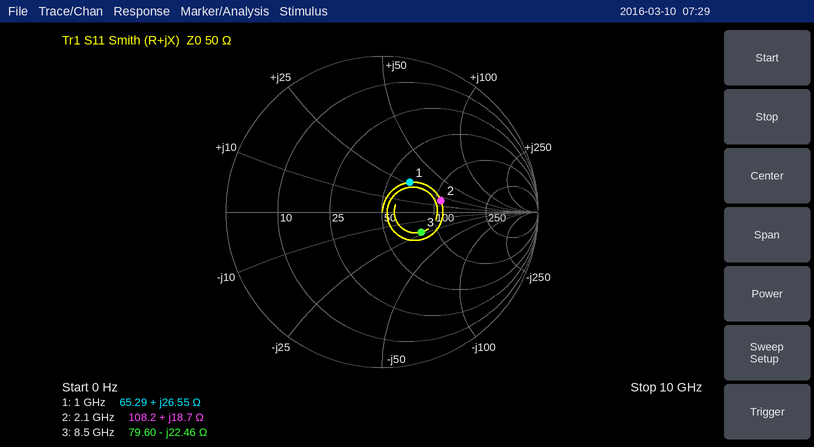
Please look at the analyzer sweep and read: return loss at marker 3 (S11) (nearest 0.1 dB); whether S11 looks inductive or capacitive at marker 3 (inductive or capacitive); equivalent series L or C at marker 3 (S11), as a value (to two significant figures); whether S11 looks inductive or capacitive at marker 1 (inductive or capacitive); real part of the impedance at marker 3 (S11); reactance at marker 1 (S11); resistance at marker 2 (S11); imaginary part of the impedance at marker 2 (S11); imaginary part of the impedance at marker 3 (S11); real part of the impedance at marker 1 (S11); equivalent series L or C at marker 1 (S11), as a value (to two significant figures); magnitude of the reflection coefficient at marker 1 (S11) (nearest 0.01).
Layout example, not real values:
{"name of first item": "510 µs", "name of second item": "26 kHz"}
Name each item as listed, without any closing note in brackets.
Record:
{"return loss at marker 3 (S11)": "11.0 dB", "whether S11 looks inductive or capacitive at marker 3": "capacitive", "equivalent series L or C at marker 3 (S11), as a value": "830 fF", "whether S11 looks inductive or capacitive at marker 1": "inductive", "real part of the impedance at marker 3": "79.60 Ω", "reactance at marker 1": "+26.55 Ω", "resistance at marker 2": "108.2 Ω", "imaginary part of the impedance at marker 2": "+18.7 Ω", "imaginary part of the impedance at marker 3": "-22.46 Ω", "real part of the impedance at marker 1": "65.29 Ω", "equivalent series L or C at marker 1 (S11), as a value": "4.2 nH", "magnitude of the reflection coefficient at marker 1 (S11)": "0.26"}
